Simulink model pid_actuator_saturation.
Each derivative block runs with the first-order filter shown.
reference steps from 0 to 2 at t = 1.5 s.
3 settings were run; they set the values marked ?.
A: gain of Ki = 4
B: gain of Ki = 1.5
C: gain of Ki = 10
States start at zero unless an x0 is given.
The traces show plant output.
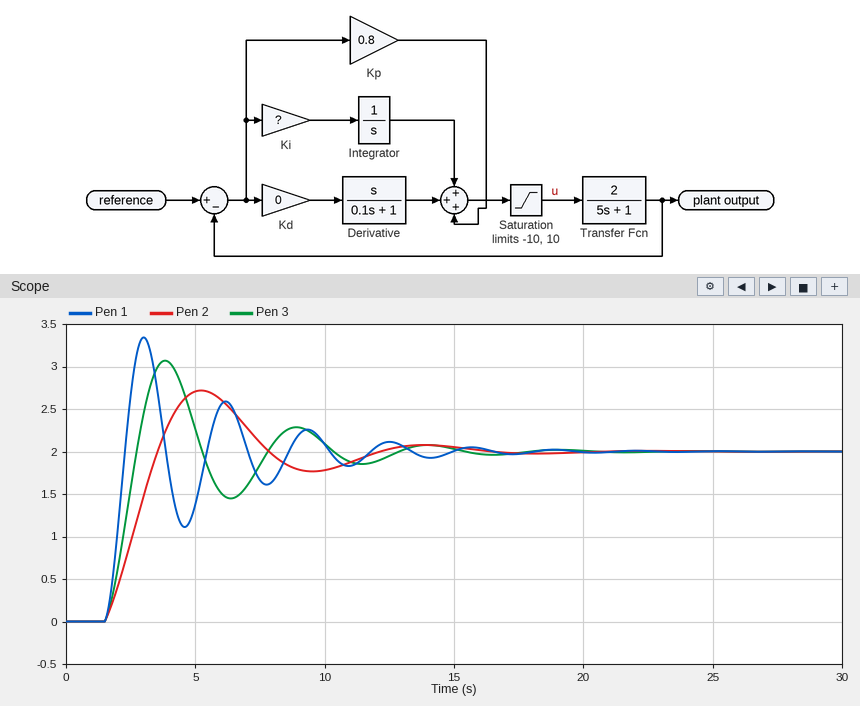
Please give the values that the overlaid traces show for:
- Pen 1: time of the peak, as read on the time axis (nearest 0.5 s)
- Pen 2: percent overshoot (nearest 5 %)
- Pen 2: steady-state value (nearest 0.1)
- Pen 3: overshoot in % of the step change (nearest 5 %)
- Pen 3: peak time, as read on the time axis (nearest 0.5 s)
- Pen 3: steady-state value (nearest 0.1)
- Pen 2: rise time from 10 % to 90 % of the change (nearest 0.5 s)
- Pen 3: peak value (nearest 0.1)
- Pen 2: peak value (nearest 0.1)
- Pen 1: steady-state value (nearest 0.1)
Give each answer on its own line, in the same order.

3.0 s
35 %
2.0
55 %
4.0 s
2.0
1.5 s
3.1
2.7
2.0
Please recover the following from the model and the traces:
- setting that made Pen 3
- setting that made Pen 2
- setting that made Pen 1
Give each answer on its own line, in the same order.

A
B
C
